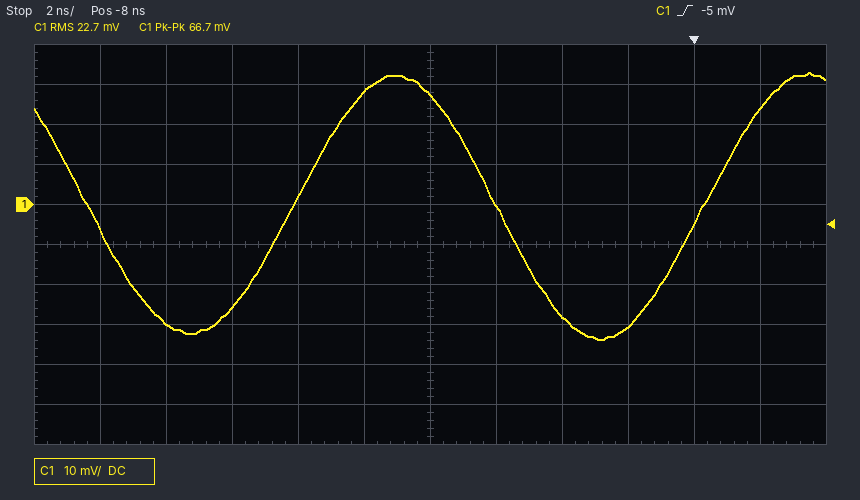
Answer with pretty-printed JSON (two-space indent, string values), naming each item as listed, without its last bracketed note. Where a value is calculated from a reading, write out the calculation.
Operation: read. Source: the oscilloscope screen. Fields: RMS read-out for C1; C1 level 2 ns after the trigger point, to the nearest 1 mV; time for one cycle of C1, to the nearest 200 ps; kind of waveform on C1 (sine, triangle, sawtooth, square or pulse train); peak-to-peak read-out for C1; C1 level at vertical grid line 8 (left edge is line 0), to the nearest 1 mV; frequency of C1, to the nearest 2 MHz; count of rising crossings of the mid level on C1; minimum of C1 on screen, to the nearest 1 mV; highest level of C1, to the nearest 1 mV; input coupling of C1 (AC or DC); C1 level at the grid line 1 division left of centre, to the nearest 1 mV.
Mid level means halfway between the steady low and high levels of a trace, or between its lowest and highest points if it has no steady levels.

{
  "RMS read-out for C1": "22.7 mV",
  "C1 level 2 ns after the trigger point, to the nearest 1 mV": "24 mV",
  "time for one cycle of C1, to the nearest 200 ps": "12.4 ns",
  "kind of waveform on C1": "sine",
  "peak-to-peak read-out for C1": "66.7 mV",
  "C1 level at vertical grid line 8 (left edge is line 0), to the nearest 1 mV": "-28 mV",
  "frequency of C1, to the nearest 2 MHz": "1 / 12.4 ns ≈ 80.6 MHz, so 80 MHz to the nearest 2 MHz",
  "count of rising crossings of the mid level on C1": "2",
  "minimum of C1 on screen, to the nearest 1 mV": "-34 mV",
  "highest level of C1, to the nearest 1 mV": "33 mV",
  "input coupling of C1": "DC",
  "C1 level at the grid line 1 division left of centre, to the nearest 1 mV": "28 mV"
}
